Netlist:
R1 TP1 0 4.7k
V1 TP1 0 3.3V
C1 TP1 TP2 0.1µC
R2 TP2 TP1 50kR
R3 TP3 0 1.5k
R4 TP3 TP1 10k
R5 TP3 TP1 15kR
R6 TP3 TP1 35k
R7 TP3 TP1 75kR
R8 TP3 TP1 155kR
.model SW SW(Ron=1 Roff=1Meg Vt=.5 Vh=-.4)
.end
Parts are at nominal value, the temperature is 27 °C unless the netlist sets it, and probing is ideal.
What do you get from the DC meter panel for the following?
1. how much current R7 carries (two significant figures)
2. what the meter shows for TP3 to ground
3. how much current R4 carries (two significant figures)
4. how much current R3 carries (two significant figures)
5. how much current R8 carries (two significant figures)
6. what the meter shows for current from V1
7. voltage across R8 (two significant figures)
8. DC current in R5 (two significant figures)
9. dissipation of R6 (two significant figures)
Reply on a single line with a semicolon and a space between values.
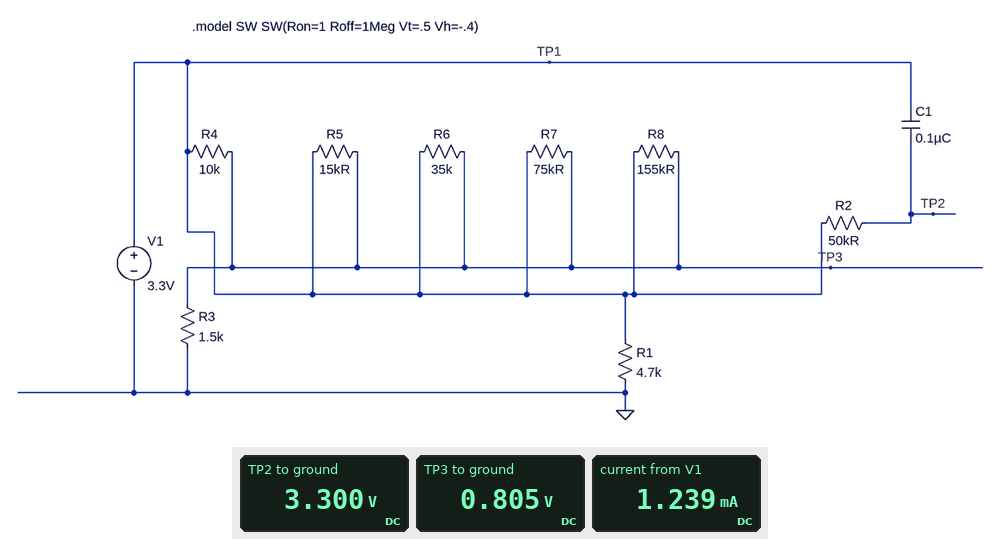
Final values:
33 µA; 0.805 V; 250 µA; 540 µA; 16 µA; 1.239 mA; 2.5 V; 170 µA; 180 µW
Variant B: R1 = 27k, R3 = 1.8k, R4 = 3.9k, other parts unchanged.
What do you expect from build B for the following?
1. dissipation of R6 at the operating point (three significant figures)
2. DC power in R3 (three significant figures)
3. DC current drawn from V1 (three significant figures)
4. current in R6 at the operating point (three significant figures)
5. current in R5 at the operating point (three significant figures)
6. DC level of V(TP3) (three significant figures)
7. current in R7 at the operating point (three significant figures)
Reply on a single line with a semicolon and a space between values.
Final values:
112 µW; 971 µW; 857 µA; 56.5 µA; 132 µA; 1.32 V; 26.4 µA
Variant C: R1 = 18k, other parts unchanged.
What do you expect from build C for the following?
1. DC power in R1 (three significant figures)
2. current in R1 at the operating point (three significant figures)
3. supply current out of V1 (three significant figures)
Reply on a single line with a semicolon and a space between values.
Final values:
605 µW; 183 µA; 720 µA
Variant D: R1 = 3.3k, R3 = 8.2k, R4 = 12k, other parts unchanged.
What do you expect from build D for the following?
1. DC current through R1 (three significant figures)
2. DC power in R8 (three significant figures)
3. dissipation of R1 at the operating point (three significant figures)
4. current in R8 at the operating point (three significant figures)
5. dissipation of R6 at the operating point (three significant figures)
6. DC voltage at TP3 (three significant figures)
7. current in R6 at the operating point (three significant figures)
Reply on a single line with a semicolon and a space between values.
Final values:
1.00 mA; 10.2 µW; 3.30 mW; 8.11 µA; 45.1 µW; 2.04 V; 35.9 µA
